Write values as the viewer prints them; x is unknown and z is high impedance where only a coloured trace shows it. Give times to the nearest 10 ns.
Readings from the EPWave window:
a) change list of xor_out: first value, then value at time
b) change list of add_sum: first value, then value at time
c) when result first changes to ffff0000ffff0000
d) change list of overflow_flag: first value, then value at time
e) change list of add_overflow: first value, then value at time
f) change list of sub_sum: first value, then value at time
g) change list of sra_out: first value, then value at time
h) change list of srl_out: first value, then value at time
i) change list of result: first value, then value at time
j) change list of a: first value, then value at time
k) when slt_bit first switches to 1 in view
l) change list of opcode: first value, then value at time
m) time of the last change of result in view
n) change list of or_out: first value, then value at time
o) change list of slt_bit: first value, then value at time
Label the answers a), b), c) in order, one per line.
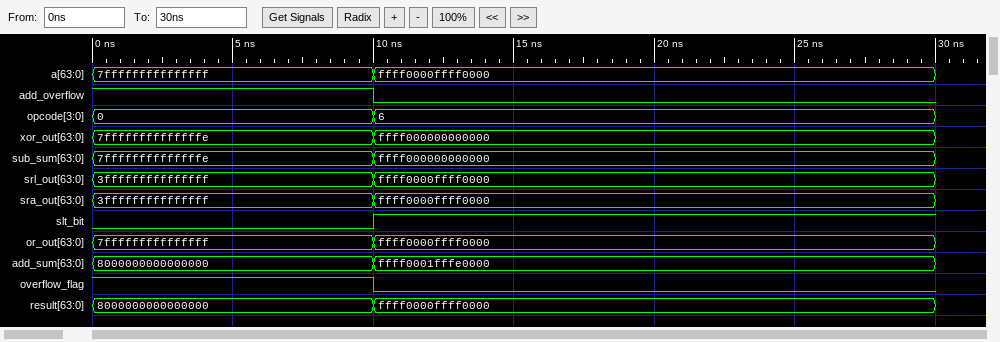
a) 7ffffffffffffffe, ffff000000000000 at 10 ns
b) 8000000000000000, ffff0001fffe0000 at 10 ns
c) 10 ns
d) 1, 0 at 10 ns
e) 1, 0 at 10 ns
f) 7ffffffffffffffe, ffff000000000000 at 10 ns
g) 3fffffffffffffff, ffff0000ffff0000 at 10 ns
h) 3fffffffffffffff, ffff0000ffff0000 at 10 ns
i) 8000000000000000, ffff0000ffff0000 at 10 ns
j) 7fffffffffffffff, ffff0000ffff0000 at 10 ns
k) 10 ns
l) 0, 6 at 10 ns
m) 10 ns
n) 7fffffffffffffff, ffff0000ffff0000 at 10 ns
o) 0, 1 at 10 ns
